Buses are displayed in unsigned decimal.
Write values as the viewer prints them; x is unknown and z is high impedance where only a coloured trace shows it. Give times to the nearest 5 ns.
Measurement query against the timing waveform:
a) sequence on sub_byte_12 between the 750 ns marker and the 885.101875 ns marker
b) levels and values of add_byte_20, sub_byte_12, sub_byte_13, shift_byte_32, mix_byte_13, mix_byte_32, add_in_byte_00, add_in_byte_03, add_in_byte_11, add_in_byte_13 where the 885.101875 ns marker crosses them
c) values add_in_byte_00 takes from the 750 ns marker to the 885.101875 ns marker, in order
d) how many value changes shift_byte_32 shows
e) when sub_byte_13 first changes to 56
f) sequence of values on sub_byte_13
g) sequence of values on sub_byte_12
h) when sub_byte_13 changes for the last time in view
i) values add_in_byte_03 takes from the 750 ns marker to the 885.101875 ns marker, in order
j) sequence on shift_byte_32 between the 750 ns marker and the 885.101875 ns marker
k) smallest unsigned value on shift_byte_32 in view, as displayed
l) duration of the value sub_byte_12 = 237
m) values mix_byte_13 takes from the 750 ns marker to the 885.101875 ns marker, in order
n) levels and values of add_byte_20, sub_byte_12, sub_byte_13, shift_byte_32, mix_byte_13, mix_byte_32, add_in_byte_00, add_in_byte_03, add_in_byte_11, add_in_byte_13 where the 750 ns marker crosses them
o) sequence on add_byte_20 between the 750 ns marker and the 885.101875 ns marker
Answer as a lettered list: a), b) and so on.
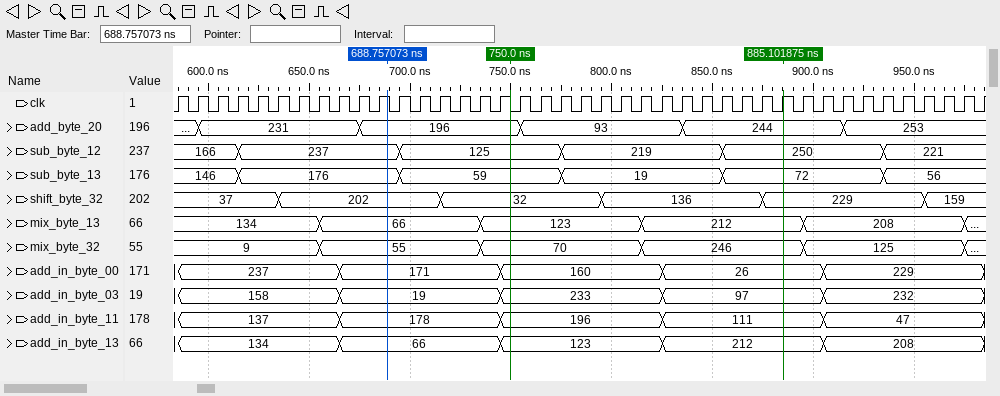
a) 125, 219, 250
b) add_byte_20=244, sub_byte_12=250, sub_byte_13=72, shift_byte_32=229, mix_byte_13=212, mix_byte_32=246, add_in_byte_00=26, add_in_byte_03=97, add_in_byte_11=111, add_in_byte_13=212
c) 160, 26
d) 5
e) 935 ns
f) 146, 176, 59, 19, 72, 56
g) 166, 237, 125, 219, 250, 221
h) 935 ns
i) 233, 97
j) 32, 136, 229
k) 32
l) 80 ns
m) 123, 212
n) add_byte_20=196, sub_byte_12=125, sub_byte_13=59, shift_byte_32=32, mix_byte_13=123, mix_byte_32=70, add_in_byte_00=160, add_in_byte_03=233, add_in_byte_11=196, add_in_byte_13=123
o) 196, 93, 244
